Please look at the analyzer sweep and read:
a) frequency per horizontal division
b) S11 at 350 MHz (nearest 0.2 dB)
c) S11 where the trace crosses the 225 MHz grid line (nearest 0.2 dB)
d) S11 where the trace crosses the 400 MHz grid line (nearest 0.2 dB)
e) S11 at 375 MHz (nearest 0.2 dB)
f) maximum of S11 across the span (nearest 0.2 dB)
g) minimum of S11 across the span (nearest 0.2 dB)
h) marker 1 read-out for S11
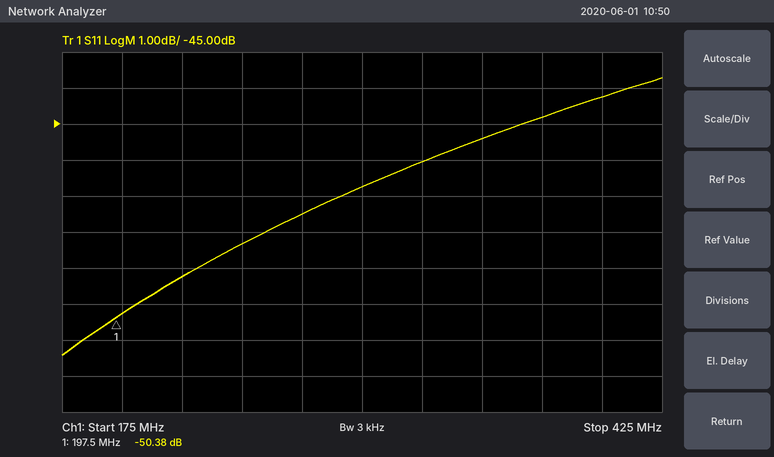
25 MHz
-45.4 dB
-49.2 dB
-44.2 dB
-44.8 dB
-43.8 dB
-51.4 dB
-50.38 dB
